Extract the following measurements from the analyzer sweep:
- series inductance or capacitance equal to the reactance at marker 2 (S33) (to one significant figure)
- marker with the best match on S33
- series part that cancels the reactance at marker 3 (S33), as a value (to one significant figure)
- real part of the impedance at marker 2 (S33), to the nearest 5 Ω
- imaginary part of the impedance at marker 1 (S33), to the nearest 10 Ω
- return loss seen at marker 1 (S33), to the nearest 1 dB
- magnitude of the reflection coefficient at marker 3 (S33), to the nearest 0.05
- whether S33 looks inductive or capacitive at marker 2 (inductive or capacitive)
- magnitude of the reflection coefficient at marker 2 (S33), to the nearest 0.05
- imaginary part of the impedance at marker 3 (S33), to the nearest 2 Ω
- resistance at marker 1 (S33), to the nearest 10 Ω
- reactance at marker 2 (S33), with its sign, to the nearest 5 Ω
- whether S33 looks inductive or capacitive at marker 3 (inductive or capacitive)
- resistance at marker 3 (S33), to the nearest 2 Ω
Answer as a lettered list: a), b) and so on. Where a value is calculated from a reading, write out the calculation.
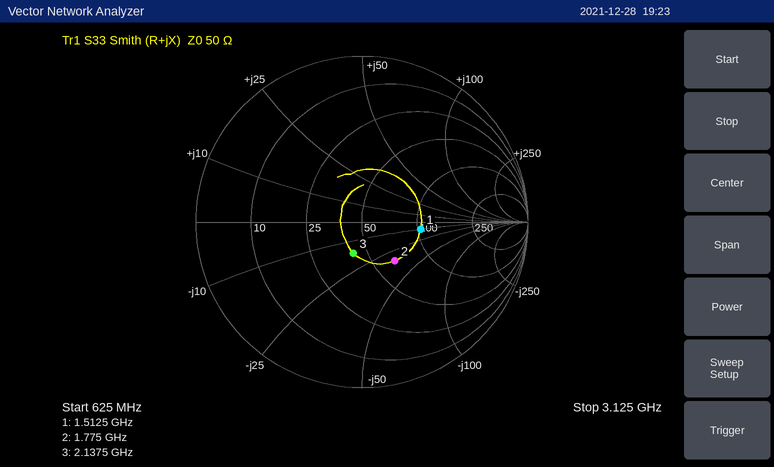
a) C = 1/(2π × 1.775 GHz × 35 Ω) ≈ 3 pF
b) marker 3
c) L = 16 Ω/(2π × 2.1375 GHz) ≈ 1 nH
d) 65 Ω
e) -10 Ω
f) 9 dB
g) 0.20
h) capacitive
i) 0.30
j) -16 Ω
k) 100 Ω
l) -35 Ω
m) capacitive
n) 42 Ω
